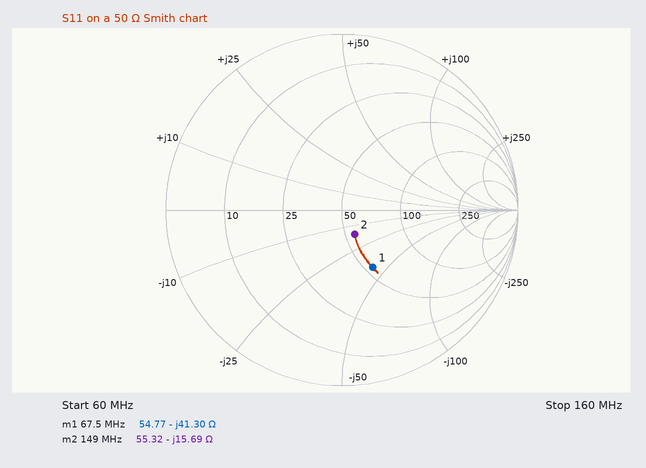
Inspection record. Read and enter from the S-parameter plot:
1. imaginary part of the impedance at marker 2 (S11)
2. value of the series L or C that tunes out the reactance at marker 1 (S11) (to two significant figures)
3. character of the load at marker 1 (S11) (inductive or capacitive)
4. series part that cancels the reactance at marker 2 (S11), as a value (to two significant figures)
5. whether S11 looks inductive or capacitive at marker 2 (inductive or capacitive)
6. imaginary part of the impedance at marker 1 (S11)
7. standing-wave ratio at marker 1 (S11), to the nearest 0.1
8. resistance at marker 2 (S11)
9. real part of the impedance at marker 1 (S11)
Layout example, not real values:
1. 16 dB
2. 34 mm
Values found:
1. -15.69 Ω
2. 97 nH
3. capacitive
4. 17 nH
5. capacitive
6. -41.30 Ω
7. 2.2
8. 55.32 Ω
9. 54.77 Ω
